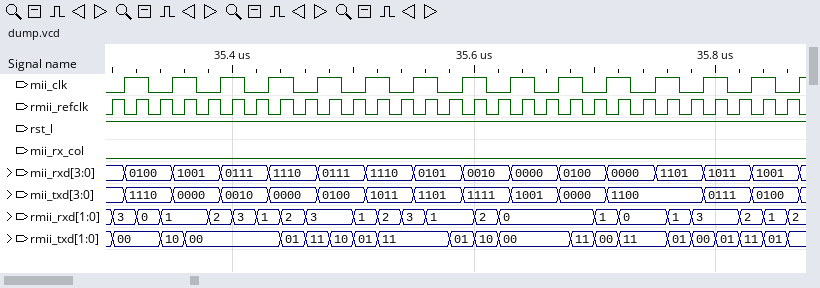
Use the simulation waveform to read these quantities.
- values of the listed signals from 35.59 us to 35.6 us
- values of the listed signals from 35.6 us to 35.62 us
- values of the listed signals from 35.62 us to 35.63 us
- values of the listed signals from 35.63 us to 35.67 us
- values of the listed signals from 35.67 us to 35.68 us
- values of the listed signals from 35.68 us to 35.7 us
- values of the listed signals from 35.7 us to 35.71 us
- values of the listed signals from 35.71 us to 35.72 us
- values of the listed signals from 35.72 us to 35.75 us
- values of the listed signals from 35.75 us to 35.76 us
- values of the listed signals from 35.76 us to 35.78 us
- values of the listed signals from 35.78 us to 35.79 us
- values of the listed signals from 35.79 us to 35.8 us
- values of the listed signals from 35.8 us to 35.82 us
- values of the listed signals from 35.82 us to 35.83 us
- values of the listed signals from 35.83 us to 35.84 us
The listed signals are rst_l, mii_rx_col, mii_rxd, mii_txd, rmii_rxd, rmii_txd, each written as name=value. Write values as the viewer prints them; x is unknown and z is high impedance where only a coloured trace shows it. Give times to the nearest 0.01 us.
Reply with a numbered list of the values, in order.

1. rst_l=1, mii_rx_col=0, mii_rxd=0010, mii_txd=1111, rmii_rxd=1, rmii_txd=01
2. rst_l=1, mii_rx_col=0, mii_rxd=0010, mii_txd=1111, rmii_rxd=2, rmii_txd=10
3. rst_l=1, mii_rx_col=0, mii_rxd=0010, mii_txd=1111, rmii_rxd=0, rmii_txd=00
4. rst_l=1, mii_rx_col=0, mii_rxd=0000, mii_txd=1001, rmii_rxd=0, rmii_txd=00
5. rst_l=1, mii_rx_col=0, mii_rxd=0100, mii_txd=0000, rmii_rxd=0, rmii_txd=00
6. rst_l=1, mii_rx_col=0, mii_rxd=0100, mii_txd=0000, rmii_rxd=0, rmii_txd=11
7. rst_l=1, mii_rx_col=0, mii_rxd=0100, mii_txd=0000, rmii_rxd=1, rmii_txd=00
8. rst_l=1, mii_rx_col=0, mii_rxd=0000, mii_txd=1100, rmii_rxd=1, rmii_txd=00
9. rst_l=1, mii_rx_col=0, mii_rxd=0000, mii_txd=1100, rmii_rxd=0, rmii_txd=11
10. rst_l=1, mii_rx_col=0, mii_rxd=1101, mii_txd=1100, rmii_rxd=0, rmii_txd=11
11. rst_l=1, mii_rx_col=0, mii_rxd=1101, mii_txd=1100, rmii_rxd=1, rmii_txd=01
12. rst_l=1, mii_rx_col=0, mii_rxd=1101, mii_txd=1100, rmii_rxd=3, rmii_txd=00
13. rst_l=1, mii_rx_col=0, mii_rxd=1011, mii_txd=0111, rmii_rxd=3, rmii_txd=00
14. rst_l=1, mii_rx_col=0, mii_rxd=1011, mii_txd=0111, rmii_rxd=3, rmii_txd=01
15. rst_l=1, mii_rx_col=0, mii_rxd=1011, mii_txd=0111, rmii_rxd=2, rmii_txd=11
16. rst_l=1, mii_rx_col=0, mii_rxd=1001, mii_txd=0100, rmii_rxd=2, rmii_txd=11
